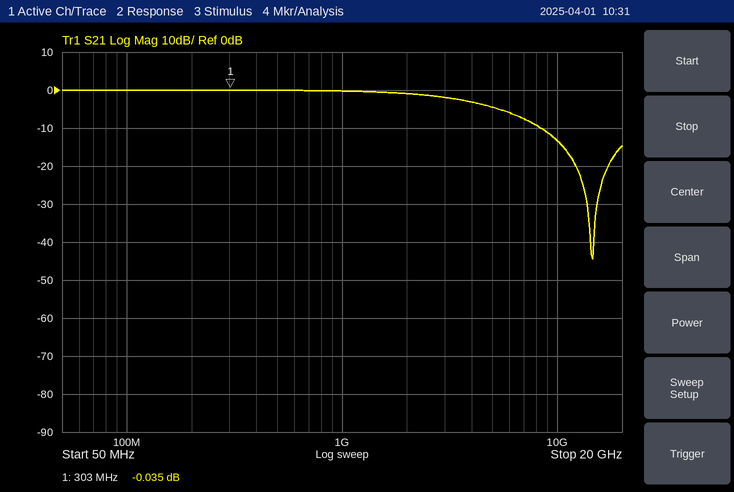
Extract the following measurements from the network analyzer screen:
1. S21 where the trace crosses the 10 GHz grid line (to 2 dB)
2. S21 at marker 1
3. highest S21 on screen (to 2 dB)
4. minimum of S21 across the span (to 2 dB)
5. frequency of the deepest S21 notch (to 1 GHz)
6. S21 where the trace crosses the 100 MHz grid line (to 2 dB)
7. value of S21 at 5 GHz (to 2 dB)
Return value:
-14 dB
-0.035 dB
0 dB
-44 dB
15 GHz
0 dB
-4 dB
